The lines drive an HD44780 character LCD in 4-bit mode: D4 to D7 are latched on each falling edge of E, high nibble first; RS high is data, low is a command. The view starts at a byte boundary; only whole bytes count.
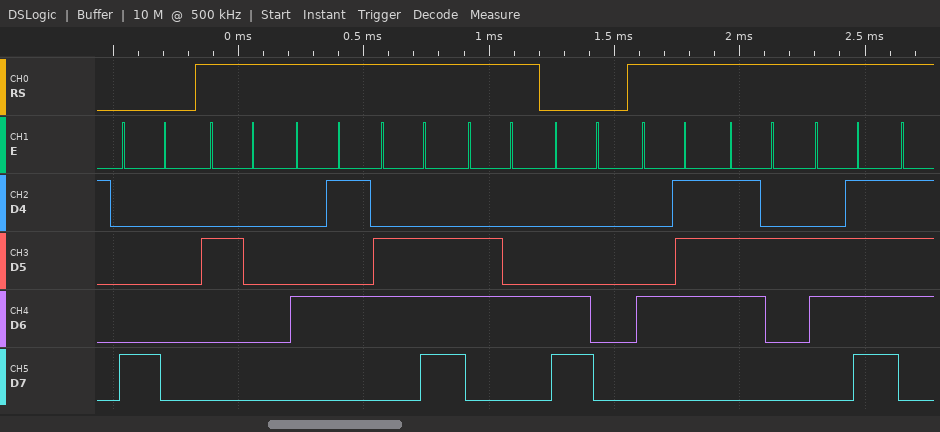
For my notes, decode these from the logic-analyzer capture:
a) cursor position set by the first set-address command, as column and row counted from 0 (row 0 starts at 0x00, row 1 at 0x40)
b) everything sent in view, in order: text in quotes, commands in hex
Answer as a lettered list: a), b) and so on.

a) column 0, row 0
b) 0x80 " End" 0xC0 "Gro"
